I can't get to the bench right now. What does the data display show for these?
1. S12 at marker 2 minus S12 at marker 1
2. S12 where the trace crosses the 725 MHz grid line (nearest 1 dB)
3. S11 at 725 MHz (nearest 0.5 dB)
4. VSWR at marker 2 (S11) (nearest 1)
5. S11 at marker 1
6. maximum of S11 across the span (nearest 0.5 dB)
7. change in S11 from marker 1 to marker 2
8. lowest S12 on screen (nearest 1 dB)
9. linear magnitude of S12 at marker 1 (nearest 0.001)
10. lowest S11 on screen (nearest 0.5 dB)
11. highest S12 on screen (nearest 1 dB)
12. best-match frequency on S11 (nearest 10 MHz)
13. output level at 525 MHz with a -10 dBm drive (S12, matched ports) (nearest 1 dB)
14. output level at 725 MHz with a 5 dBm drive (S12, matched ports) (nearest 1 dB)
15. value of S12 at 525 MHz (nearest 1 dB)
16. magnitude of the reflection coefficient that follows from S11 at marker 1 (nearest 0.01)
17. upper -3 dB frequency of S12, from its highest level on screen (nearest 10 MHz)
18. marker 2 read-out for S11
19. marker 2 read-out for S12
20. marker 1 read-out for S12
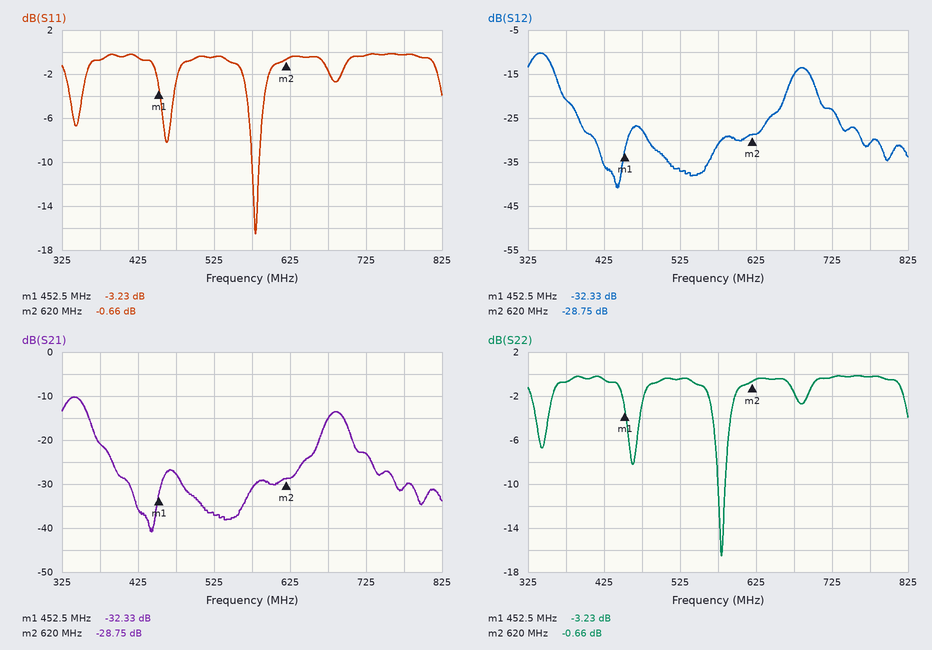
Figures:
3.58 dB
-23 dB
-0.5 dB
26
-3.23 dB
0.0 dB
2.57 dB
-41 dB
0.024
-16.5 dB
-10 dB
580 MHz
-47 dBm
-18 dBm
-37 dB
0.69
360 MHz
-0.66 dB
-28.75 dB
-32.33 dB
